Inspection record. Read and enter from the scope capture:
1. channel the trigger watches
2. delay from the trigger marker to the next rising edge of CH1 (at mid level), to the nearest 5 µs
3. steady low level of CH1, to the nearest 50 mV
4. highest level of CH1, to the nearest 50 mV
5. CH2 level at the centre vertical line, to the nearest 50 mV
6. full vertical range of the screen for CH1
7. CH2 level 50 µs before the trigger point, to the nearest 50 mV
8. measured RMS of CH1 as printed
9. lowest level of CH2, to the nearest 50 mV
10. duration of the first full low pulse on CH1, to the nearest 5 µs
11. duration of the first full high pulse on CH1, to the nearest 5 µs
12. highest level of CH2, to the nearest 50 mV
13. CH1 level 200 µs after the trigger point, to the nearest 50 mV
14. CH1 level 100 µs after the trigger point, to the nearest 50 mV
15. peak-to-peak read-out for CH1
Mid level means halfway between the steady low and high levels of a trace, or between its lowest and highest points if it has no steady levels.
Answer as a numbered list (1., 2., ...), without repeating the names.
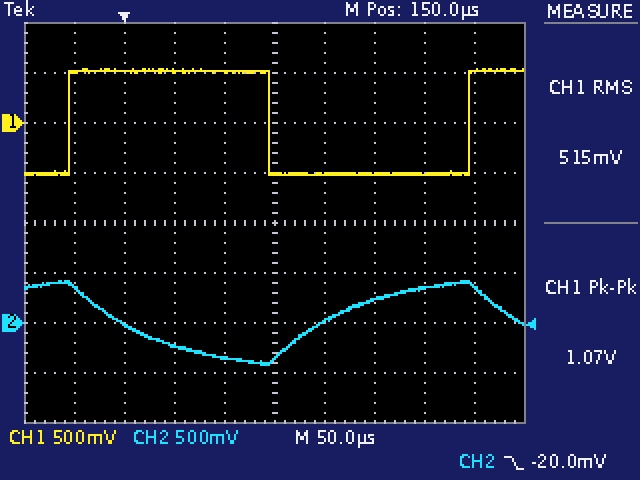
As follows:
1. CH2
2. 345 µs
3. -500 mV
4. 550 mV
5. -350 mV
6. 4 V
7. 350 mV
8. 515 mV
9. -400 mV
10. 200 µs
11. 200 µs
12. 400 mV
13. -500 mV
14. 500 mV
15. 1.07 V
